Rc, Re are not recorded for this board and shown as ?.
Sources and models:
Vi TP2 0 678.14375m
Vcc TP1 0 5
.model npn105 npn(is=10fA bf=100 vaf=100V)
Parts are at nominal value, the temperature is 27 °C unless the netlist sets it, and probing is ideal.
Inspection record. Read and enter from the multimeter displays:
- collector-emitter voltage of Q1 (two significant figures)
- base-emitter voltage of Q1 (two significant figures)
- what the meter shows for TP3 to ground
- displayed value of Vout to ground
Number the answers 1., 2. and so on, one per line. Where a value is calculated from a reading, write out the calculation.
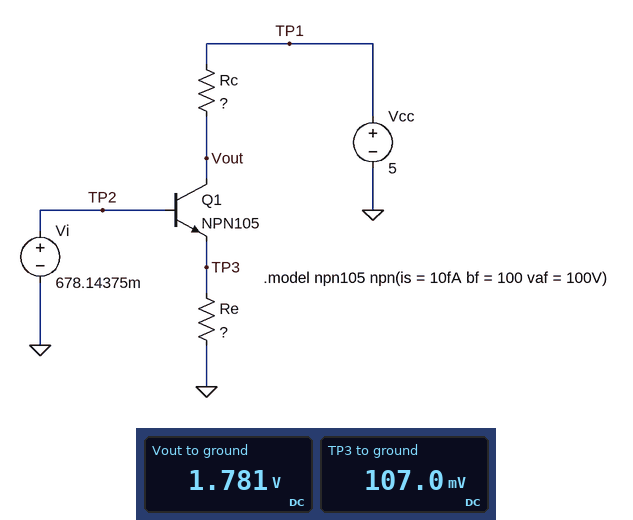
1. 1.781 V - 107 mV = 1.7 V
2. 678.1 mV - 107 mV = 570 mV
3. 107.0 mV
4. 1.781 V
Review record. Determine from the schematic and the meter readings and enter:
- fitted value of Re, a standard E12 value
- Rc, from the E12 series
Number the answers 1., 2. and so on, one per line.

1. 2.7 kΩ
2. 82 kΩ
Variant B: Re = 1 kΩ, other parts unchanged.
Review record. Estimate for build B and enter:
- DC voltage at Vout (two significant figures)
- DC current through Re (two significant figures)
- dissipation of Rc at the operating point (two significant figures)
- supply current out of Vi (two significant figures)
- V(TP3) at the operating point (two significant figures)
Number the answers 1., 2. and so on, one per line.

1. 120 mV
2. 82 µA
3. 290 µW
4. 22 µA
5. 82 mV
